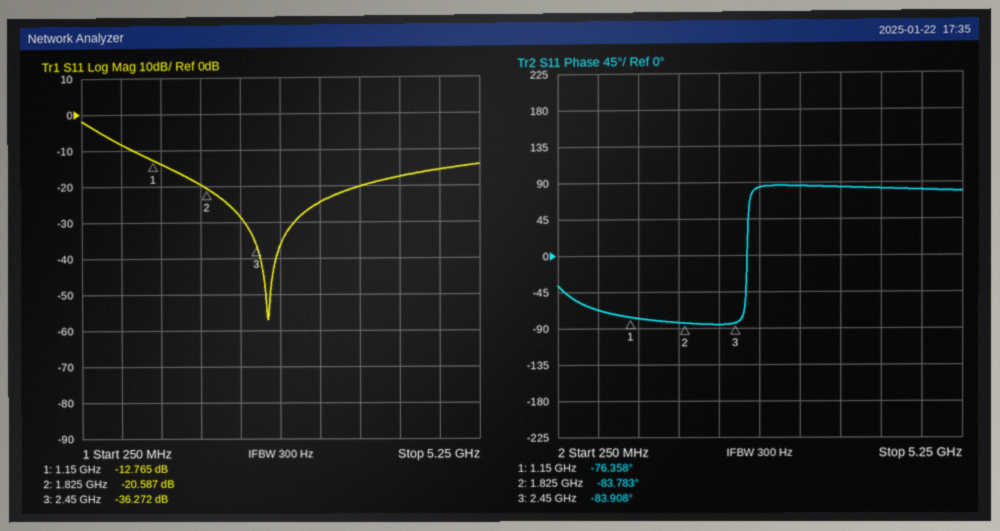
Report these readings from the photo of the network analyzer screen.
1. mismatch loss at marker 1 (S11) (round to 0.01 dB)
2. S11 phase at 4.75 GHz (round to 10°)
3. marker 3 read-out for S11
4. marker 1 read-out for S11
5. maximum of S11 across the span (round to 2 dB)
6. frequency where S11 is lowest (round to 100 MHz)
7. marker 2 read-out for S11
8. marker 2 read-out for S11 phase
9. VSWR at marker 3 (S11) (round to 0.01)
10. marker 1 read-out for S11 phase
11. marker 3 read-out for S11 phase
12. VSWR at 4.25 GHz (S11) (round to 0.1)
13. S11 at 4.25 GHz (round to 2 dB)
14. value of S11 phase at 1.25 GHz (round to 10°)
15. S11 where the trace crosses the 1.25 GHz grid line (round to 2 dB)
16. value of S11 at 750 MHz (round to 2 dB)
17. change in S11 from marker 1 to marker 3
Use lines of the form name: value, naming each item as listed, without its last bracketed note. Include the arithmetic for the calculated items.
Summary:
mismatch loss at marker 1 (S11): −10 log10(1 − 10^(-12.765/10)) ≈ 0.24 dB
S11 phase at 4.75 GHz: 80°
marker 3 read-out for S11: -36.272 dB
marker 1 read-out for S11: -12.765 dB
maximum of S11 across the span: -2 dB
frequency where S11 is lowest: 2.6 GHz
marker 2 read-out for S11: -20.587 dB
marker 2 read-out for S11 phase: -83.783°
VSWR at marker 3 (S11): (1 + 0.0154)/(1 − 0.0154) ≈ 1.03
marker 1 read-out for S11 phase: -76.358°
marker 3 read-out for S11 phase: -83.908°
VSWR at 4.25 GHz (S11): |Γ| = 10^(-18/20) = 0.1259; VSWR = (1 + 0.1259)/(1 − 0.1259) ≈ 1.3
S11 at 4.25 GHz: -18 dB
value of S11 phase at 1.25 GHz: -80°
S11 where the trace crosses the 1.25 GHz grid line: -14 dB
value of S11 at 750 MHz: -8 dB
change in S11 from marker 1 to marker 3: -36.272 − (-12.765) = -23.507 dB
